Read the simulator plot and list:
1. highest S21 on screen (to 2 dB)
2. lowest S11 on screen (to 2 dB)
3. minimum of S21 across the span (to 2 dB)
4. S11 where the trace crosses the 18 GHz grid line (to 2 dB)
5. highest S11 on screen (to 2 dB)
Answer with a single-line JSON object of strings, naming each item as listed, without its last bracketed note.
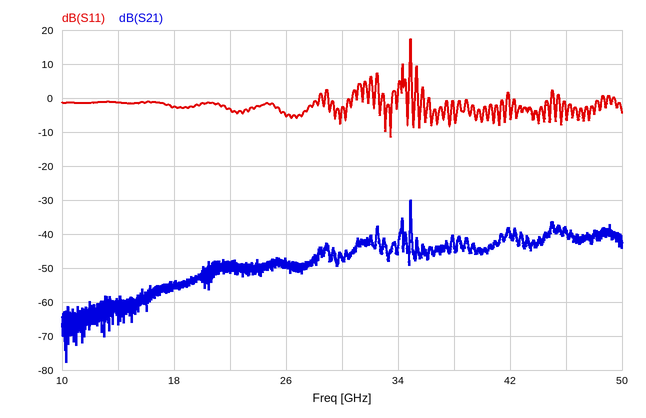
{"highest S21 on screen": "-30 dB", "lowest S11 on screen": "-12 dB", "minimum of S21 across the span": "-78 dB", "S11 where the trace crosses the 18 GHz grid line": "-2 dB", "highest S11 on screen": "18 dB"}
